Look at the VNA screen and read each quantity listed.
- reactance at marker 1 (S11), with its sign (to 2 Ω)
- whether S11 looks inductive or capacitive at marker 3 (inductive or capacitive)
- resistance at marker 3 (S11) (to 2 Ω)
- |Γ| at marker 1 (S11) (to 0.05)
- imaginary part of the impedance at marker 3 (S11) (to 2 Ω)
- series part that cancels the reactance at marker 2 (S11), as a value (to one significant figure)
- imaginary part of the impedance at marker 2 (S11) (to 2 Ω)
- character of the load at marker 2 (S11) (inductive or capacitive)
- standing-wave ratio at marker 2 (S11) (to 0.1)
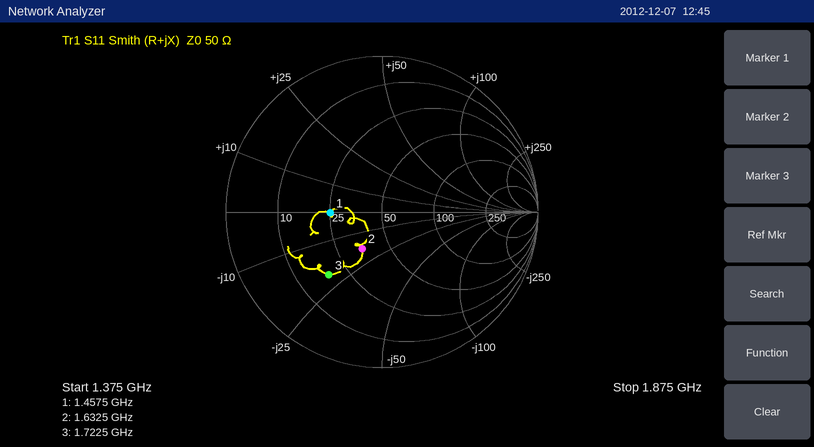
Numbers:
0 Ω
capacitive
18 Ω
0.35
-20 Ω
2 nH
-18 Ω
capacitive
1.7
